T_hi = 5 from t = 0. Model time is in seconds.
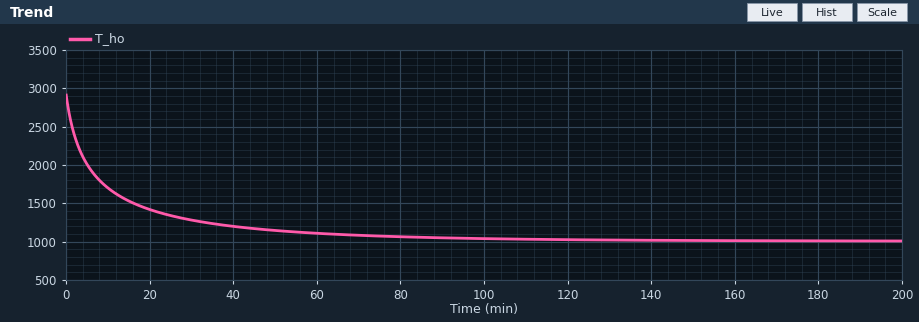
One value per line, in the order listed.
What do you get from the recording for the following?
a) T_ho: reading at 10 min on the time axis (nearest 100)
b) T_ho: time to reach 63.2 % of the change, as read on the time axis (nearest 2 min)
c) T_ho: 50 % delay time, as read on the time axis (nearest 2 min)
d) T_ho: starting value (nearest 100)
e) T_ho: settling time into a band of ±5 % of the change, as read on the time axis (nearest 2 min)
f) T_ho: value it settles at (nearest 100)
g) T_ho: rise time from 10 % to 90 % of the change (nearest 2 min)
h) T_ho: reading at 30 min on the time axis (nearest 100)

1700
10 min
6 min
2900
62 min
1000
40 min
1300
